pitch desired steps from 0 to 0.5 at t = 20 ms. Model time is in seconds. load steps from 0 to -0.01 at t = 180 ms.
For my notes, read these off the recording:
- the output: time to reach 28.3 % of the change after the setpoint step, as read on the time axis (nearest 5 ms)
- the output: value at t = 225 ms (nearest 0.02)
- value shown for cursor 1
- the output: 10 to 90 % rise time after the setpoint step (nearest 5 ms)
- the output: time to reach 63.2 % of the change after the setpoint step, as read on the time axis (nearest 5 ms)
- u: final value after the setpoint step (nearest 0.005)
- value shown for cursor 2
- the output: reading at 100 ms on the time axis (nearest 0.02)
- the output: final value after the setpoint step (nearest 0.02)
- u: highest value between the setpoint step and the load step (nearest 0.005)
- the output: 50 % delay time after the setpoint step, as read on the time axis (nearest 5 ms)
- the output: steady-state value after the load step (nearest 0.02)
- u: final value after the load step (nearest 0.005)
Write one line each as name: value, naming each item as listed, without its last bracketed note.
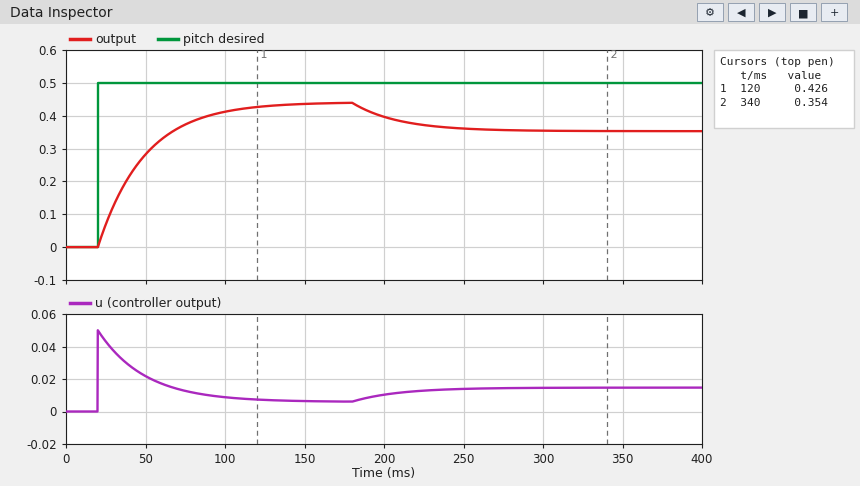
the output: time to reach 28.3 % of the change after the setpoint step, as read on the time axis: 30 ms
the output: value at t = 225 ms: 0.38
value shown for cursor 1: 0.426
the output: 10 to 90 % rise time after the setpoint step: 65 ms
the output: time to reach 63.2 % of the change after the setpoint step, as read on the time axis: 50 ms
u: final value after the setpoint step: 0.005
value shown for cursor 2: 0.354
the output: reading at 100 ms on the time axis: 0.42
the output: final value after the setpoint step: 0.44
u: highest value between the setpoint step and the load step: 0.050
the output: 50 % delay time after the setpoint step, as read on the time axis: 40 ms
the output: steady-state value after the load step: 0.36
u: final value after the load step: 0.015
